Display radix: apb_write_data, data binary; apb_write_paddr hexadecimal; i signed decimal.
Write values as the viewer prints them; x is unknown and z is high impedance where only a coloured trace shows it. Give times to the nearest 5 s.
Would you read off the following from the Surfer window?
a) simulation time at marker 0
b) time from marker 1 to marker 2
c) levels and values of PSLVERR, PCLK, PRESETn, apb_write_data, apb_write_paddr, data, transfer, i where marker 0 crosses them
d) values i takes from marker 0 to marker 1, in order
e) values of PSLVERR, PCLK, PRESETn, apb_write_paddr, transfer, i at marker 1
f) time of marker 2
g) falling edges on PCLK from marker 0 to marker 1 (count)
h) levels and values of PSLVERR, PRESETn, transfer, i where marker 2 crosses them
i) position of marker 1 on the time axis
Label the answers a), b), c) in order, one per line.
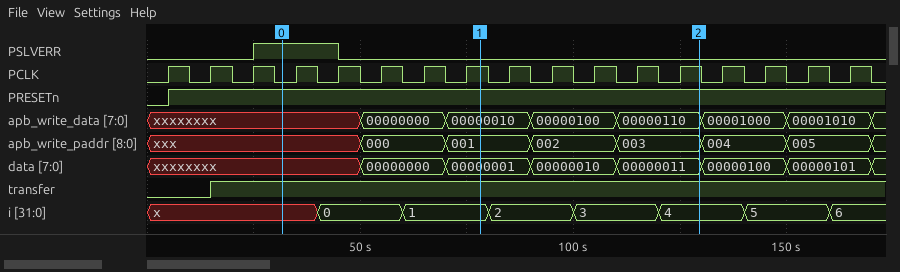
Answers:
a) 30 s
b) 50 s
c) PSLVERR=1, PCLK=0, PRESETn=1, apb_write_data=xxxxxxxx, apb_write_paddr=xxx, data=xxxxxxxx, transfer=1, i=x
d) x, 0, 1
e) PSLVERR=0, PCLK=1, PRESETn=1, apb_write_paddr=001, transfer=1, i=1
f) 130 s
g) 4
h) PSLVERR=0, PRESETn=1, transfer=1, i=4
i) 80 s
